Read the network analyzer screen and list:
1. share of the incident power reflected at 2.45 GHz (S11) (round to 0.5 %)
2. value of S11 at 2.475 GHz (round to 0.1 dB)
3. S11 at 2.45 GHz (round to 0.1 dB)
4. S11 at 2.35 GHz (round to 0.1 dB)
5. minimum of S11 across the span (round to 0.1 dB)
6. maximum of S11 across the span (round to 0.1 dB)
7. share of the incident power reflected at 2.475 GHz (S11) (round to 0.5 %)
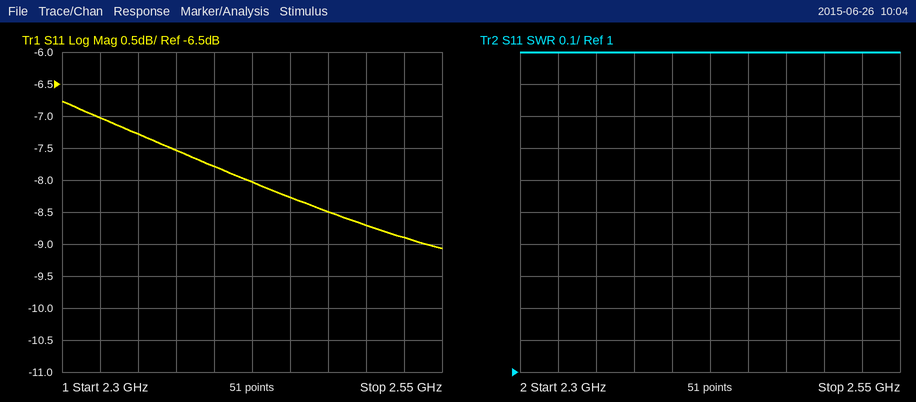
15.0 %
-8.5 dB
-8.3 dB
-7.3 dB
-9.1 dB
-6.8 dB
14.0 %
